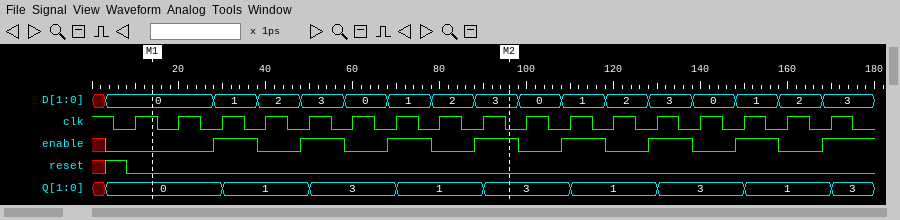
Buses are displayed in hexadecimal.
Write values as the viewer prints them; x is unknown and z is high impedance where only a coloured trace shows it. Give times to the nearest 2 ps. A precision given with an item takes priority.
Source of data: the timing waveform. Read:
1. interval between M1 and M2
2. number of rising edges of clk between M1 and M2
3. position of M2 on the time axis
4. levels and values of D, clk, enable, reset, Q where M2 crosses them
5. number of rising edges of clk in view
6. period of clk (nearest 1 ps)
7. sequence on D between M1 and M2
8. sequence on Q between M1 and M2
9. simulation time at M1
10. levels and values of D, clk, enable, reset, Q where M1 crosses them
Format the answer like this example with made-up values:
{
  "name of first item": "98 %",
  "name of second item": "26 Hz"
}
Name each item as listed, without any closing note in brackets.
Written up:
{
  "interval between M1 and M2": "82 ps",
  "number of rising edges of clk between M1 and M2": "8",
  "position of M2 on the time axis": "96 ps",
  "levels and values of D, clk, enable, reset, Q where M2 crosses them": "D=3, clk=0, enable=1, reset=0, Q=3",
  "number of rising edges of clk in view": "17",
  "period of clk": "10 ps",
  "sequence on D between M1 and M2": "0, 1, 2, 3, 0, 1, 2, 3",
  "sequence on Q between M1 and M2": "0, 1, 3, 1, 3",
  "simulation time at M1": "14 ps",
  "levels and values of D, clk, enable, reset, Q where M1 crosses them": "D=0, clk=1, enable=0, reset=0, Q=0"
}
